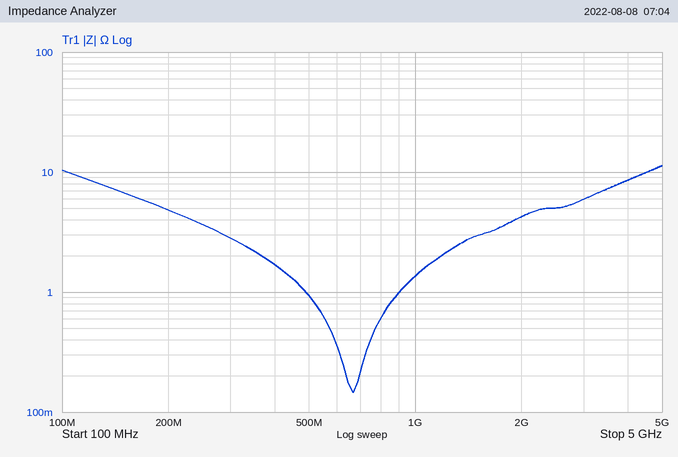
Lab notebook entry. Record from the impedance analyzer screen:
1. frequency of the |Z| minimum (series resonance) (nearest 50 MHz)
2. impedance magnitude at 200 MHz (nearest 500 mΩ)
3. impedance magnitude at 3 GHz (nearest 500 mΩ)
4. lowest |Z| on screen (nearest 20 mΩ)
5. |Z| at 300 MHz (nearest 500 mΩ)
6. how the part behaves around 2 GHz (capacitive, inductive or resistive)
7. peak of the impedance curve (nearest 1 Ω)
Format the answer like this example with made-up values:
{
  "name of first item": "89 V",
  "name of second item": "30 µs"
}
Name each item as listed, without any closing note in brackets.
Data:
{
  "frequency of the |Z| minimum (series resonance)": "650 MHz",
  "impedance magnitude at 200 MHz": "5.0 Ω",
  "impedance magnitude at 3 GHz": "6.0 Ω",
  "lowest |Z| on screen": "140 mΩ",
  "|Z| at 300 MHz": "3.0 Ω",
  "how the part behaves around 2 GHz": "inductive",
  "peak of the impedance curve": "11 Ω"
}
